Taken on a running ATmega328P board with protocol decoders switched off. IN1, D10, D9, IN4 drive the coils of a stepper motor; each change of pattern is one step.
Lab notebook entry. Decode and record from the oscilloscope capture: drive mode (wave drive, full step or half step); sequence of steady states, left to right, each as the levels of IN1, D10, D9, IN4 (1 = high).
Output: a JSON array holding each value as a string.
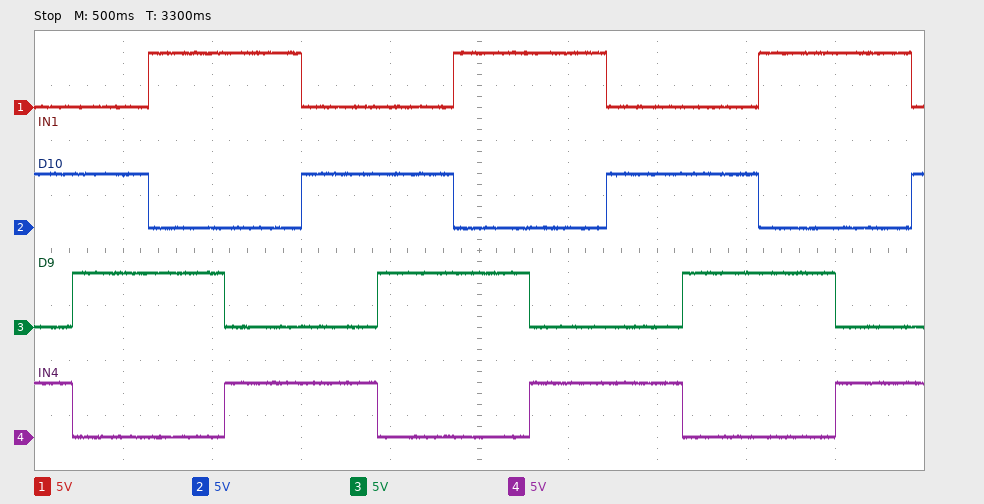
["full step", "0101 0110 1010 1001 0101 0110 1010 1001 0101 0110 1010 1001 0101"]
